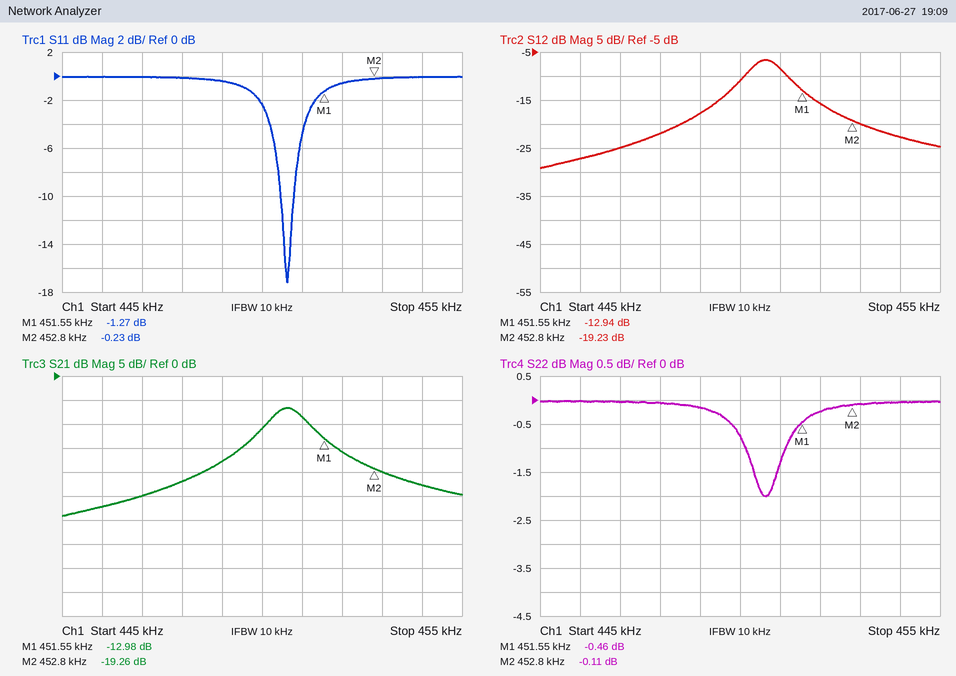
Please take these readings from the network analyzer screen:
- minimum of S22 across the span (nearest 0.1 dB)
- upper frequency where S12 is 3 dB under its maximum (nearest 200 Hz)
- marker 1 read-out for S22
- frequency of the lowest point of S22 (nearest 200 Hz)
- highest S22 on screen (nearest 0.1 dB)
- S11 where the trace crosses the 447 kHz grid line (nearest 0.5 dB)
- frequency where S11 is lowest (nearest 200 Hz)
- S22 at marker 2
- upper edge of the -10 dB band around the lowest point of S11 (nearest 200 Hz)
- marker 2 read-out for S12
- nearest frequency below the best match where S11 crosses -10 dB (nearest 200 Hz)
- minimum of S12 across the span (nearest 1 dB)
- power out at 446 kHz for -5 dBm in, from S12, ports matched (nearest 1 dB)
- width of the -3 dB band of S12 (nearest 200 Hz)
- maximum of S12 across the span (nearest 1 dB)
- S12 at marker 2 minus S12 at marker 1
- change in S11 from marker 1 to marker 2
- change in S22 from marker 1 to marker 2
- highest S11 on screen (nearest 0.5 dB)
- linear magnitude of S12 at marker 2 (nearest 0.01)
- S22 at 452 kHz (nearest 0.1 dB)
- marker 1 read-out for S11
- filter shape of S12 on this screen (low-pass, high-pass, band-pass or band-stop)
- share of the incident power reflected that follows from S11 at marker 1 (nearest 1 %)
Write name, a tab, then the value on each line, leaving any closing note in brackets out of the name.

minimum of S22 across the span	-2.0 dB
upper frequency where S12 is 3 dB under its maximum	451.2 kHz
marker 1 read-out for S22	-0.46 dB
frequency of the lowest point of S22	450.6 kHz
highest S22 on screen	0.0 dB
S11 where the trace crosses the 447 kHz grid line	0.0 dB
frequency where S11 is lowest	450.6 kHz
S22 at marker 2	-0.11 dB
upper edge of the -10 dB band around the lowest point of S11	450.8 kHz
marker 2 read-out for S12	-19.23 dB
nearest frequency below the best match where S11 crosses -10 dB	450.4 kHz
minimum of S12 across the span	-29 dB
power out at 446 kHz for -5 dBm in, from S12, ports matched	-32 dBm
width of the -3 dB band of S12	1.0 kHz
maximum of S12 across the span	-7 dB
S12 at marker 2 minus S12 at marker 1	-6.29 dB
change in S11 from marker 1 to marker 2	1.04 dB
change in S22 from marker 1 to marker 2	0.35 dB
highest S11 on screen	0.0 dB
linear magnitude of S12 at marker 2	0.11
S22 at 452 kHz	-0.2 dB
marker 1 read-out for S11	-1.27 dB
filter shape of S12 on this screen	band-pass
share of the incident power reflected that follows from S11 at marker 1	75 %
